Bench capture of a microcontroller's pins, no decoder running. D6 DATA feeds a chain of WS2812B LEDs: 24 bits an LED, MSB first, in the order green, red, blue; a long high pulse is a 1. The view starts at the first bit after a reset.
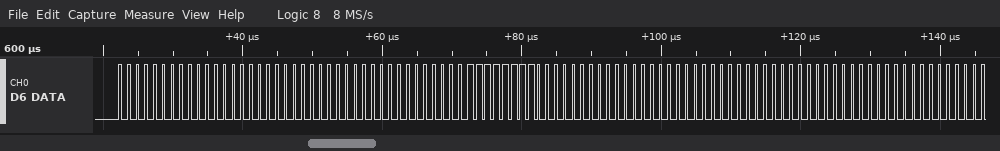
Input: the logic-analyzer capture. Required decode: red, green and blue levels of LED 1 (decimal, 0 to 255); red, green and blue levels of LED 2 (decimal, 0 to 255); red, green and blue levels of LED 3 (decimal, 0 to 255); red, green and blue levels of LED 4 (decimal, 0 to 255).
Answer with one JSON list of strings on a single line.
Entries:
["0, 0, 0", "0, 0, 255", "0, 0, 0", "0, 0, 0"]
